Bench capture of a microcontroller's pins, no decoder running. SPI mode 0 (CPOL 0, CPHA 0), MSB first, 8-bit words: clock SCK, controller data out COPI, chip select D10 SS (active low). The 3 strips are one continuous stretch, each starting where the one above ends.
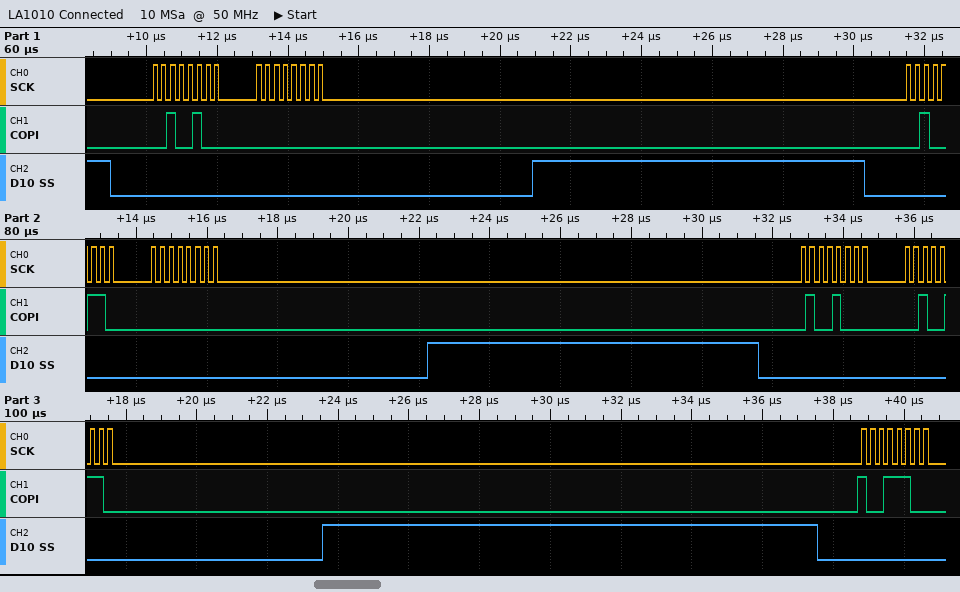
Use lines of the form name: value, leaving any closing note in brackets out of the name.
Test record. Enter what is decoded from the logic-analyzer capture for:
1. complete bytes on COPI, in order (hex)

complete bytes on COPI, in order: 0x24 0x00 0x26 0x00 0x48 0x26 0x9C
